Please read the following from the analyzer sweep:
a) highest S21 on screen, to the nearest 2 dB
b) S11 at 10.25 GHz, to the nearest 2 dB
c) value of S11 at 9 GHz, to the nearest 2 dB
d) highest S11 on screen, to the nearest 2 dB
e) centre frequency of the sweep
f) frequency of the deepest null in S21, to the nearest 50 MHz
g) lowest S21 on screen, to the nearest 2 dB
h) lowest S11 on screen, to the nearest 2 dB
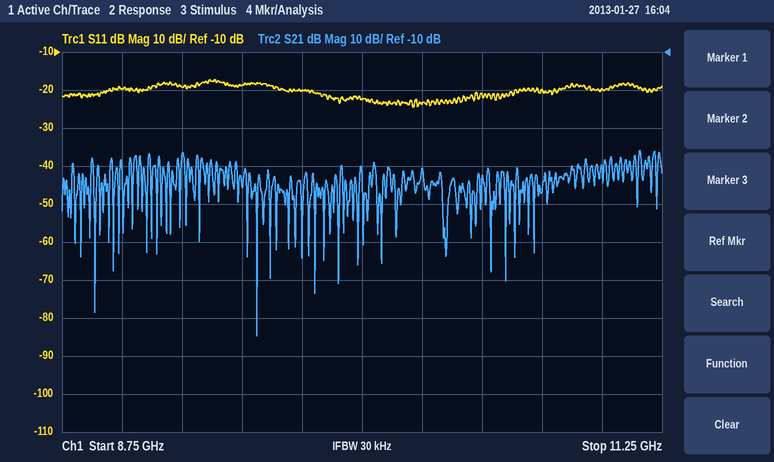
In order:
-36 dB
-24 dB
-20 dB
-18 dB
10 GHz
9.55 GHz
-84 dB
-24 dB
